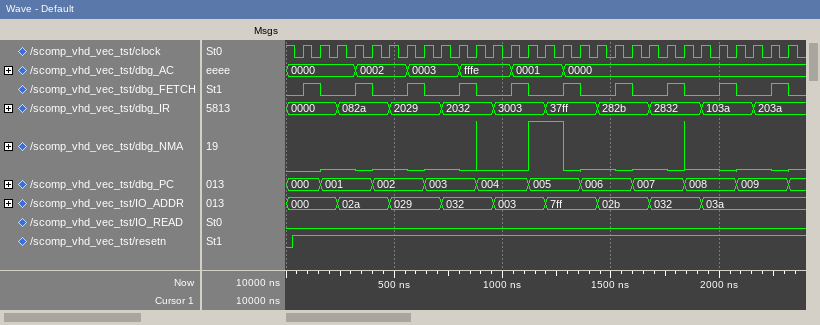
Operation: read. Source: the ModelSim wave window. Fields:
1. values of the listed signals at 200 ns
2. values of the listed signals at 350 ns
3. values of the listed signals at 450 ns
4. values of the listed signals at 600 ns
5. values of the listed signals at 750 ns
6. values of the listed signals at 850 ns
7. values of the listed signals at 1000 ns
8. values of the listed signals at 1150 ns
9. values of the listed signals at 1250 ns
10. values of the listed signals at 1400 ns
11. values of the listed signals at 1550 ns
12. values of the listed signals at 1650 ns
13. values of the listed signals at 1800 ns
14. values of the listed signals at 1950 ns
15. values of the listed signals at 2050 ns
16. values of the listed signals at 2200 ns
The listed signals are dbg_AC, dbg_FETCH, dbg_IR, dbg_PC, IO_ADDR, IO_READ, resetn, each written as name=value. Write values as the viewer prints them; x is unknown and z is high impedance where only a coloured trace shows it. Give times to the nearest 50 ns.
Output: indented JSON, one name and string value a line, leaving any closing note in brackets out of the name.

{
  "values of the listed signals at 200 ns": "dbg_AC=0000, dbg_FETCH=0, dbg_IR=0000, dbg_PC=001, IO_ADDR=000, IO_READ=0, resetn=1",
  "values of the listed signals at 350 ns": "dbg_AC=0002, dbg_FETCH=1, dbg_IR=082a, dbg_PC=001, IO_ADDR=02a, IO_READ=0, resetn=1",
  "values of the listed signals at 450 ns": "dbg_AC=0002, dbg_FETCH=0, dbg_IR=082a, dbg_PC=002, IO_ADDR=02a, IO_READ=0, resetn=1",
  "values of the listed signals at 600 ns": "dbg_AC=0003, dbg_FETCH=1, dbg_IR=2029, dbg_PC=002, IO_ADDR=029, IO_READ=0, resetn=1",
  "values of the listed signals at 750 ns": "dbg_AC=0003, dbg_FETCH=0, dbg_IR=2032, dbg_PC=003, IO_ADDR=032, IO_READ=0, resetn=1",
  "values of the listed signals at 850 ns": "dbg_AC=fffe, dbg_FETCH=1, dbg_IR=2032, dbg_PC=003, IO_ADDR=032, IO_READ=0, resetn=1",
  "values of the listed signals at 1000 ns": "dbg_AC=fffe, dbg_FETCH=0, dbg_IR=3003, dbg_PC=004, IO_ADDR=003, IO_READ=0, resetn=1",
  "values of the listed signals at 1150 ns": "dbg_AC=0001, dbg_FETCH=0, dbg_IR=3003, dbg_PC=005, IO_ADDR=003, IO_READ=0, resetn=1",
  "values of the listed signals at 1250 ns": "dbg_AC=0001, dbg_FETCH=0, dbg_IR=37ff, dbg_PC=005, IO_ADDR=7ff, IO_READ=0, resetn=1",
  "values of the listed signals at 1400 ns": "dbg_AC=0000, dbg_FETCH=0, dbg_IR=37ff, dbg_PC=006, IO_ADDR=7ff, IO_READ=0, resetn=1",
  "values of the listed signals at 1550 ns": "dbg_AC=0000, dbg_FETCH=1, dbg_IR=282b, dbg_PC=006, IO_ADDR=02b, IO_READ=0, resetn=1",
  "values of the listed signals at 1650 ns": "dbg_AC=0000, dbg_FETCH=0, dbg_IR=282b, dbg_PC=007, IO_ADDR=02b, IO_READ=0, resetn=1",
  "values of the listed signals at 1800 ns": "dbg_AC=0000, dbg_FETCH=1, dbg_IR=2832, dbg_PC=007, IO_ADDR=032, IO_READ=0, resetn=1",
  "values of the listed signals at 1950 ns": "dbg_AC=0000, dbg_FETCH=0, dbg_IR=103a, dbg_PC=008, IO_ADDR=03a, IO_READ=0, resetn=1",
  "values of the listed signals at 2050 ns": "dbg_AC=0000, dbg_FETCH=1, dbg_IR=103a, dbg_PC=008, IO_ADDR=03a, IO_READ=0, resetn=1",
  "values of the listed signals at 2200 ns": "dbg_AC=0000, dbg_FETCH=0, dbg_IR=203a, dbg_PC=009, IO_ADDR=03a, IO_READ=0, resetn=1"
}
